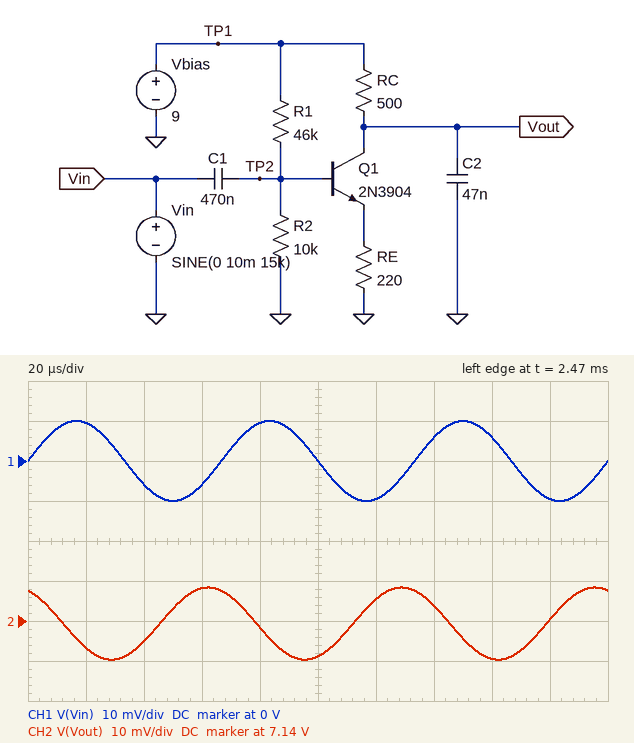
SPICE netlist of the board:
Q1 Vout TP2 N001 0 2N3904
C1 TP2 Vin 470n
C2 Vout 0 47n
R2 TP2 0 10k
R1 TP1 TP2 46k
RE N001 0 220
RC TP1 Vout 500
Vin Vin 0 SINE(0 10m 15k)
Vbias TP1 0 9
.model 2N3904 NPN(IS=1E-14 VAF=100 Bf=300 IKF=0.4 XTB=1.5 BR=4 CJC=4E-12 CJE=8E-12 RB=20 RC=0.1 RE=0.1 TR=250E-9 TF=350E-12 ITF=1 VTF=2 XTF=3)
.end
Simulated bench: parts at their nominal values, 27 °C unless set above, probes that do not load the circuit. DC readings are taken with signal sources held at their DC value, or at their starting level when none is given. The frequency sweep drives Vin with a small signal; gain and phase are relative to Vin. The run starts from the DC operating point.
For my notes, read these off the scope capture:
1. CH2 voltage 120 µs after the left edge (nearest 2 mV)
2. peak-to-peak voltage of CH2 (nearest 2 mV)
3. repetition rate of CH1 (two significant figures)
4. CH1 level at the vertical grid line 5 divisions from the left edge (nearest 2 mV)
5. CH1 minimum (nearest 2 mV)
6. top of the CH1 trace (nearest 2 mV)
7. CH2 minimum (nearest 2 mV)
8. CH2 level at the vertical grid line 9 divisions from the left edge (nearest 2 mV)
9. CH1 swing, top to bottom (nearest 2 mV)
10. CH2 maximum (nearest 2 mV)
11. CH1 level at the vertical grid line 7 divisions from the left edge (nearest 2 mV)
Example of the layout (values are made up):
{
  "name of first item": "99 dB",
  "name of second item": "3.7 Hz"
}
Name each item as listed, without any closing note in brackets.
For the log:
{
  "CH2 voltage 120 µs after the left edge": "7.146 V",
  "peak-to-peak voltage of CH2": "18 mV",
  "repetition rate of CH1": "15 kHz",
  "CH1 level at the vertical grid line 5 divisions from the left edge": "0 V",
  "CH1 minimum": "-10 mV",
  "top of the CH1 trace": "10 mV",
  "CH2 minimum": "7.130 V",
  "CH2 level at the vertical grid line 9 divisions from the left edge": "7.140 V",
  "CH1 swing, top to bottom": "20 mV",
  "CH2 maximum": "7.148 V",
  "CH1 level at the vertical grid line 7 divisions from the left edge": "6 mV"
}
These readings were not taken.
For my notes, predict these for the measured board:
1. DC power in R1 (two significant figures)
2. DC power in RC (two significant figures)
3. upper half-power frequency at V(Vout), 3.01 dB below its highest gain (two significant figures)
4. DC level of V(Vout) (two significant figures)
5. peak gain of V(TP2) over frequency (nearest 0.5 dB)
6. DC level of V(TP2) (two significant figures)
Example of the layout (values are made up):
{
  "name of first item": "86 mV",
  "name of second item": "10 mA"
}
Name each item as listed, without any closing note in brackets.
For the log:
{
  "DC power in R1": "1.2 mW",
  "DC power in RC": "6.9 mW",
  "upper half-power frequency at V(Vout), 3.01 dB below its highest gain": "6.9 kHz",
  "DC level of V(Vout)": "7.1 V",
  "peak gain of V(TP2) over frequency": "0 dB",
  "DC level of V(TP2)": "1.5 V"
}
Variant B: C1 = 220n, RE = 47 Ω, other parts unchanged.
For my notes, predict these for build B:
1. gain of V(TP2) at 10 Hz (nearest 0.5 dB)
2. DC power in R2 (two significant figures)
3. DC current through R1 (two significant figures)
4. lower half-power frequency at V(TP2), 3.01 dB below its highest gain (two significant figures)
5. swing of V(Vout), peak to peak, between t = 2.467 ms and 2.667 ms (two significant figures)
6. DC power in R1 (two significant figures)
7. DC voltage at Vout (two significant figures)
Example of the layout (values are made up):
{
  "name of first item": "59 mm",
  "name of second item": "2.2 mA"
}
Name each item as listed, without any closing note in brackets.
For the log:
{
  "gain of V(TP2) at 10 Hz": "-23.0 dB",
  "DC power in R2": "160 µW",
  "DC current through R1": "170 µA",
  "lower half-power frequency at V(TP2), 3.01 dB below its highest gain": "140 Hz",
  "swing of V(Vout), peak to peak, between t = 2.467 ms and 2.667 ms": "83 mV",
  "DC power in R1": "1.3 mW",
  "DC voltage at Vout": "3.1 V"
}
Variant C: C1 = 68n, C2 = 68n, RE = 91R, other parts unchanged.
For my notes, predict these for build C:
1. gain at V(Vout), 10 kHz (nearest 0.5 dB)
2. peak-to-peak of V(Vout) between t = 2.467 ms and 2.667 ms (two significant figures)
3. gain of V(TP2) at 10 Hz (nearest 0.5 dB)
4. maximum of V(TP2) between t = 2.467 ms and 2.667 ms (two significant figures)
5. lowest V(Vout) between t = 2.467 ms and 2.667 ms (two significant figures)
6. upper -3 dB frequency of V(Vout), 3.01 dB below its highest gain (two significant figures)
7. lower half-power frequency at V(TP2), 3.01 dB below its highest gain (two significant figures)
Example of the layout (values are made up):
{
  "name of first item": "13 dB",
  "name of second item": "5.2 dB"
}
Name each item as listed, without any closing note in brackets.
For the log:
{
  "gain at V(Vout), 10 kHz": "7.0 dB",
  "peak-to-peak of V(Vout) between t = 2.467 ms and 2.667 ms": "31 mV",
  "gain of V(TP2) at 10 Hz": "-31.5 dB",
  "maximum of V(TP2) between t = 2.467 ms and 2.667 ms": "1.4 V",
  "lowest V(Vout) between t = 2.467 ms and 2.667 ms": "5.2 V",
  "upper -3 dB frequency of V(Vout), 3.01 dB below its highest gain": "5.4 kHz",
  "lower half-power frequency at V(TP2), 3.01 dB below its highest gain": "370 Hz"
}
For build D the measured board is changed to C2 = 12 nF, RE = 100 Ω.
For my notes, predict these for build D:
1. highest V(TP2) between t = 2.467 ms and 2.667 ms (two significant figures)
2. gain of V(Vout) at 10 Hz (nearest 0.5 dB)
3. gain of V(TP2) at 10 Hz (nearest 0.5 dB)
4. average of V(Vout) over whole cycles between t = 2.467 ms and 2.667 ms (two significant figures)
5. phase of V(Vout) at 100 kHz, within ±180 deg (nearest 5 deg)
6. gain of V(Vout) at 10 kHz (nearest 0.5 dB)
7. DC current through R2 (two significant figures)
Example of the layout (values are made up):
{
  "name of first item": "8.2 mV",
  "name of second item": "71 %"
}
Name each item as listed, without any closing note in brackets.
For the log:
{
  "highest V(TP2) between t = 2.467 ms and 2.667 ms": "1.4 V",
  "gain of V(Vout) at 10 Hz": "-1.0 dB",
  "gain of V(TP2) at 10 Hz": "-14.5 dB",
  "average of V(Vout) over whole cycles between t = 2.467 ms and 2.667 ms": "5.5 V",
  "phase of V(Vout) at 100 kHz, within ±180 deg": "105 deg",
  "gain of V(Vout) at 10 kHz": "13.0 dB",
  "DC current through R2": "140 µA"
}
